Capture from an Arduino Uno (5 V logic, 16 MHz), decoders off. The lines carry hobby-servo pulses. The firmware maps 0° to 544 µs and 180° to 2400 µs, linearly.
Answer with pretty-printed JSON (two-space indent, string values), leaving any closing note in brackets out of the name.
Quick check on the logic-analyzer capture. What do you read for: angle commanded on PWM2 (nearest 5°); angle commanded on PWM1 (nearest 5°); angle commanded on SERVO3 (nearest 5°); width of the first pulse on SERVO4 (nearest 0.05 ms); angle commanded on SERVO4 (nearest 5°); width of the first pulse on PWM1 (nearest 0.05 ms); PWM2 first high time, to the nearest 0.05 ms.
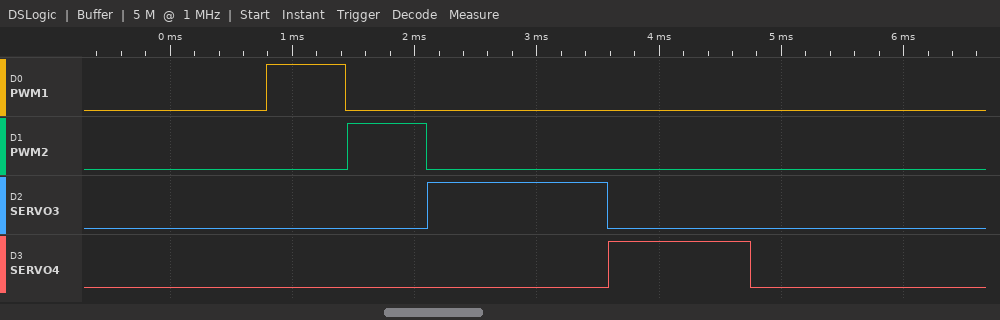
{
  "angle commanded on PWM2": "10°",
  "angle commanded on PWM1": "10°",
  "angle commanded on SERVO3": "90°",
  "width of the first pulse on SERVO4": "1.15 ms",
  "angle commanded on SERVO4": "60°",
  "width of the first pulse on PWM1": "0.65 ms",
  "PWM2 first high time, to the nearest 0.05 ms": "0.65 ms"
}
